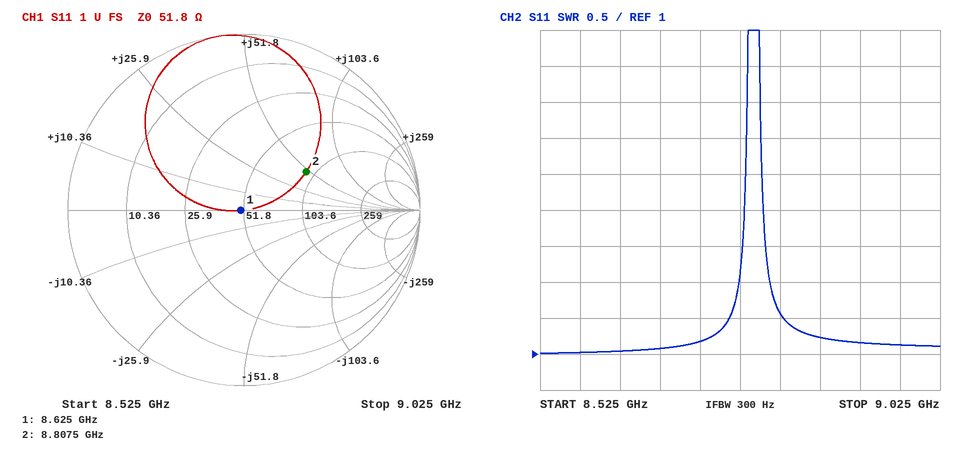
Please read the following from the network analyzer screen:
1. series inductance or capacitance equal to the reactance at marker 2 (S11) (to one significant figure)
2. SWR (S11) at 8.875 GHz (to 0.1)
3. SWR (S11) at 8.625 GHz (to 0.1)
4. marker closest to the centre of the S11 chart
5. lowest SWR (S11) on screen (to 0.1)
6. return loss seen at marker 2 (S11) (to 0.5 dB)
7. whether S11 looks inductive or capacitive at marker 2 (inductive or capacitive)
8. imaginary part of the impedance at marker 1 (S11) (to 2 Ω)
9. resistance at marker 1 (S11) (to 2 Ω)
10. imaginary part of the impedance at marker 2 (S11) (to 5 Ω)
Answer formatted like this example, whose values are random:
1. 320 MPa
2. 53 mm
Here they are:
1. 900 pH
2. 1.2
3. 1.0
4. marker 1
5. 1.0
6. 7.5 dB
7. inductive
8. 0 Ω
9. 50 Ω
10. +50 Ω
